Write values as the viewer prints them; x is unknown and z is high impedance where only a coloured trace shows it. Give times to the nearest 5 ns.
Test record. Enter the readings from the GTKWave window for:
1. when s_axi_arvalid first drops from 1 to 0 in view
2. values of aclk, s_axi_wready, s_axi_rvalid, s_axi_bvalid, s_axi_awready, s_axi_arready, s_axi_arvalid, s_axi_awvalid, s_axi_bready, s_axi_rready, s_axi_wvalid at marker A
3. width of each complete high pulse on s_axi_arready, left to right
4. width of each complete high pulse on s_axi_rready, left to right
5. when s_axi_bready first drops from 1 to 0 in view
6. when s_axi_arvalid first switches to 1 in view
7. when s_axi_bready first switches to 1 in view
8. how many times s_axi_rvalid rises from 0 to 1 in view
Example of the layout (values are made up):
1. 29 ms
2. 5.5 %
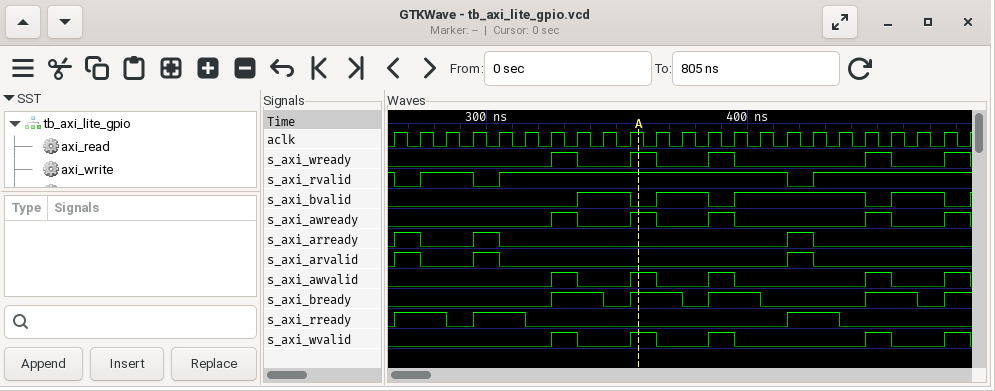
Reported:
1. 275 ns
2. aclk=1, s_axi_wready=1, s_axi_rvalid=1, s_axi_bvalid=0, s_axi_awready=1, s_axi_arready=0, s_axi_arvalid=0, s_axi_awvalid=1, s_axi_bready=1, s_axi_rready=0, s_axi_wvalid=1
3. 10 ns, 10 ns, 10 ns
4. 20 ns, 20 ns, 20 ns
5. 345 ns
6. 265 ns
7. 325 ns
8. 3
